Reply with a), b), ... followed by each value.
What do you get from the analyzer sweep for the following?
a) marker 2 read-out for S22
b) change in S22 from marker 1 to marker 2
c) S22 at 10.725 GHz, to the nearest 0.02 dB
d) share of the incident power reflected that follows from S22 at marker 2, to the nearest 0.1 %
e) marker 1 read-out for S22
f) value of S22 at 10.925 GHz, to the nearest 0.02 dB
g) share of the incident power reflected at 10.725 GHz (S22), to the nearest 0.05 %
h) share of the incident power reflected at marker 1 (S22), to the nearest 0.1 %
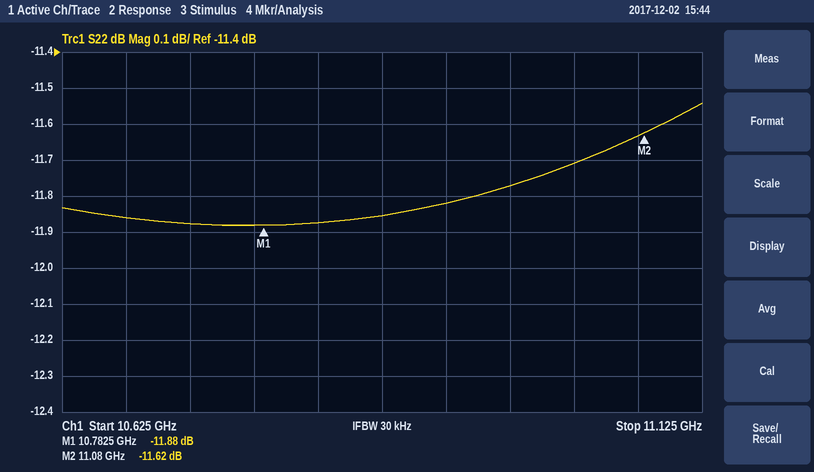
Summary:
a) -11.62 dB
b) 0.26 dB
c) -11.88 dB
d) 6.9 %
e) -11.88 dB
f) -11.82 dB
g) 6.50 %
h) 6.5 %
